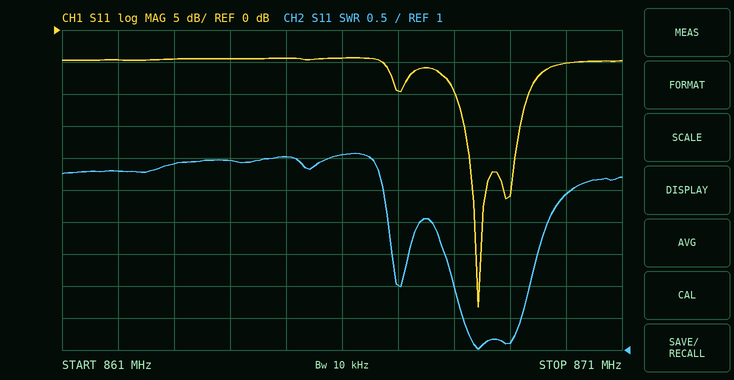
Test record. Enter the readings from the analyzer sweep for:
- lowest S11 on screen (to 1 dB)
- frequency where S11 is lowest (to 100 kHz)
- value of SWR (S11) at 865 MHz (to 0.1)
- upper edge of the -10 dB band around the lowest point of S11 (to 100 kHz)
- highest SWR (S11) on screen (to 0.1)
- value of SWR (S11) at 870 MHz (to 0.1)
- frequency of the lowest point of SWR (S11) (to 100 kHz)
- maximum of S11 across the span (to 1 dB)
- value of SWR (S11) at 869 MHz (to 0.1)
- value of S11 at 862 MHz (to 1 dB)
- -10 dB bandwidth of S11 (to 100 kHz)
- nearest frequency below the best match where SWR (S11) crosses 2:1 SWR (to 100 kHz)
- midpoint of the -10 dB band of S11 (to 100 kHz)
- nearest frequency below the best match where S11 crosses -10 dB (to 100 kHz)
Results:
-43 dB
868.4 MHz
4.0
869.3 MHz
4.1
3.4
868.4 MHz
-4 dB
1.1
-5 dB
1.3 MHz
868.0 MHz
868.7 MHz
868.0 MHz
